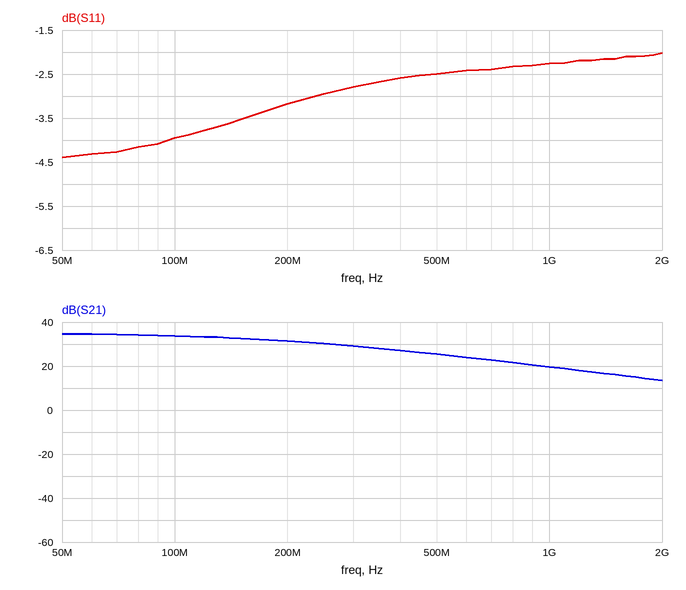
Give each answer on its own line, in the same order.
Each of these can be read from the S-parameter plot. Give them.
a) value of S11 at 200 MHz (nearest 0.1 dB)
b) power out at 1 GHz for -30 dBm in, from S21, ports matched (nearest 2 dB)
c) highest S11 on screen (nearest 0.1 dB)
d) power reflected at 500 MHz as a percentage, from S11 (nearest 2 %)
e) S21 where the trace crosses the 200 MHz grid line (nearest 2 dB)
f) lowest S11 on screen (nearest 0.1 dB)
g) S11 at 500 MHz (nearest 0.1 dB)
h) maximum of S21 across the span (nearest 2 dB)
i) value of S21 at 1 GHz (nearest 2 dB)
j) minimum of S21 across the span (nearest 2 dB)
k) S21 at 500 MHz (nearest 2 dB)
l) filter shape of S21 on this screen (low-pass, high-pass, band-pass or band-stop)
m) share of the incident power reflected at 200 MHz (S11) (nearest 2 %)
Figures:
-3.2 dB
-10 dBm
-2.0 dB
56 %
32 dB
-4.4 dB
-2.5 dB
34 dB
20 dB
14 dB
26 dB
low-pass
48 %
